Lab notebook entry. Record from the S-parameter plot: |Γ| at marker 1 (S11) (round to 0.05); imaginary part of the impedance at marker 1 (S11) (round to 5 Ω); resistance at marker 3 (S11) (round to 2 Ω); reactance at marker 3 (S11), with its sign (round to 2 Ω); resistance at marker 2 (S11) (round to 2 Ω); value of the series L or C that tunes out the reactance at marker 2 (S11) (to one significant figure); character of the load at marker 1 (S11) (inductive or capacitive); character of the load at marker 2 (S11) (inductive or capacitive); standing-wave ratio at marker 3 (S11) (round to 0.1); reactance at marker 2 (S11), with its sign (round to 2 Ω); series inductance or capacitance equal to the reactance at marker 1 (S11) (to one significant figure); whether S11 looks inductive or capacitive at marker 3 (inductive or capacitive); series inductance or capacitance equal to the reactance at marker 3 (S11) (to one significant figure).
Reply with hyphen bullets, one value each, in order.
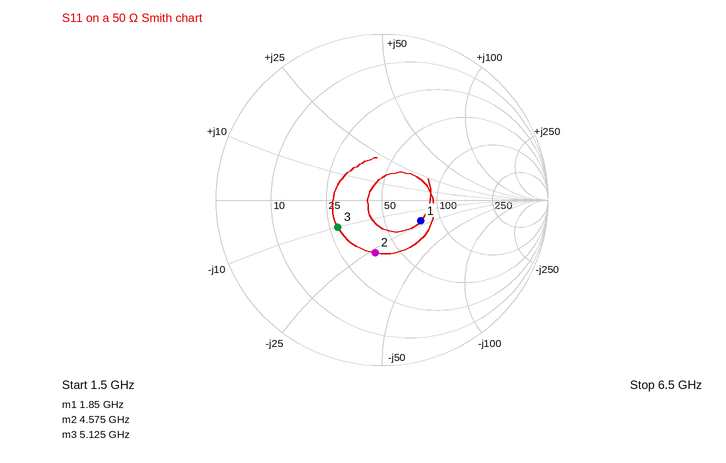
- 0.25
- -20 Ω
- 28 Ω
- -10 Ω
- 38 Ω
- 900 pH
- capacitive
- capacitive
- 1.9
- -26 Ω
- 4 pF
- capacitive
- 3 pF
